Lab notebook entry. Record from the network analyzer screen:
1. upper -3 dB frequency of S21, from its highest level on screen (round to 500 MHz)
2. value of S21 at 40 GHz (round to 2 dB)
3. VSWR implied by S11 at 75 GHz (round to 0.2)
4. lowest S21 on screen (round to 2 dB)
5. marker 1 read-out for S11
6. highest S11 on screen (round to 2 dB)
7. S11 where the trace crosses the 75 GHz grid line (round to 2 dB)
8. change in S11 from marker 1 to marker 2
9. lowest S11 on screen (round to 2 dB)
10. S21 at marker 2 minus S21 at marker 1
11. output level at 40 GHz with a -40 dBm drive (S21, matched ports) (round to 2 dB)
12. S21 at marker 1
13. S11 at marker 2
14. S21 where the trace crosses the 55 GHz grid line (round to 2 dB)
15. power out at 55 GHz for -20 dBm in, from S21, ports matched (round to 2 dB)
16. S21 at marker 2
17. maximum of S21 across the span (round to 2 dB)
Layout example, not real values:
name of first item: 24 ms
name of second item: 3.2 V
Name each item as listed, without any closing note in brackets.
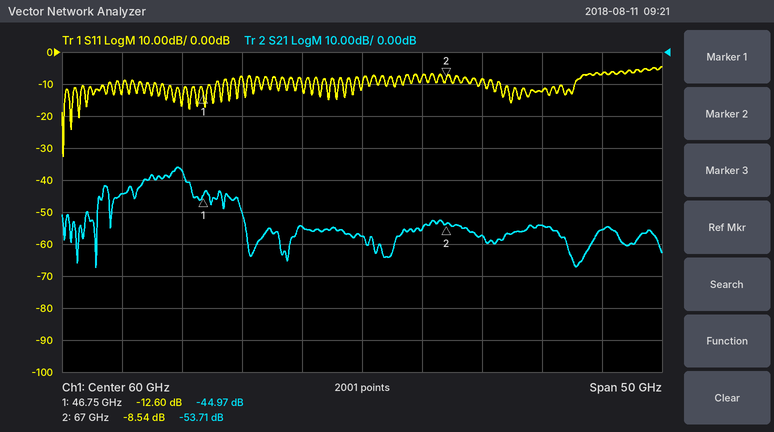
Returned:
upper -3 dB frequency of S21, from its highest level on screen: 45.0 GHz
value of S21 at 40 GHz: -44 dB
VSWR implied by S11 at 75 GHz: 1.6
lowest S21 on screen: -68 dB
marker 1 read-out for S11: -12.60 dB
highest S11 on screen: -4 dB
S11 where the trace crosses the 75 GHz grid line: -12 dB
change in S11 from marker 1 to marker 2: 4.06 dB
lowest S11 on screen: -32 dB
S21 at marker 2 minus S21 at marker 1: -8.74 dB
output level at 40 GHz with a -40 dBm drive (S21, matched ports): -84 dBm
S21 at marker 1: -44.97 dB
S11 at marker 2: -8.54 dB
S21 where the trace crosses the 55 GHz grid line: -54 dB
power out at 55 GHz for -20 dBm in, from S21, ports matched: -74 dBm
S21 at marker 2: -53.71 dB
maximum of S21 across the span: -36 dB
